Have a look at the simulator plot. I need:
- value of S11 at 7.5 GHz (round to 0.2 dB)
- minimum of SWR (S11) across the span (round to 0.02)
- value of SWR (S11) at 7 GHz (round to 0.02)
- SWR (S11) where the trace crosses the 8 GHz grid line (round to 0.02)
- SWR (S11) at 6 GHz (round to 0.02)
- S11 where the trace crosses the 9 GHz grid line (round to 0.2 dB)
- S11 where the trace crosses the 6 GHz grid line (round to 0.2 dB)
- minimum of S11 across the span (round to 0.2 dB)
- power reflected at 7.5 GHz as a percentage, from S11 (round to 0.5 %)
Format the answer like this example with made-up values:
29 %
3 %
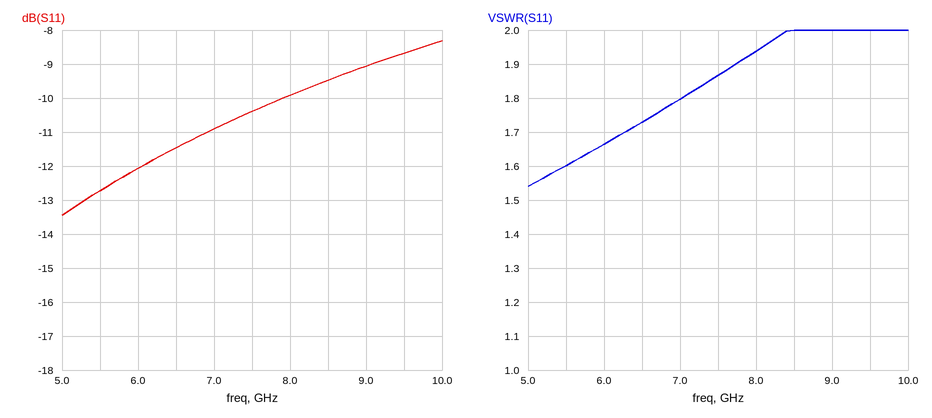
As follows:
-10.4 dB
1.54
1.80
1.94
1.66
-9.0 dB
-12.0 dB
-13.4 dB
9.0 %
